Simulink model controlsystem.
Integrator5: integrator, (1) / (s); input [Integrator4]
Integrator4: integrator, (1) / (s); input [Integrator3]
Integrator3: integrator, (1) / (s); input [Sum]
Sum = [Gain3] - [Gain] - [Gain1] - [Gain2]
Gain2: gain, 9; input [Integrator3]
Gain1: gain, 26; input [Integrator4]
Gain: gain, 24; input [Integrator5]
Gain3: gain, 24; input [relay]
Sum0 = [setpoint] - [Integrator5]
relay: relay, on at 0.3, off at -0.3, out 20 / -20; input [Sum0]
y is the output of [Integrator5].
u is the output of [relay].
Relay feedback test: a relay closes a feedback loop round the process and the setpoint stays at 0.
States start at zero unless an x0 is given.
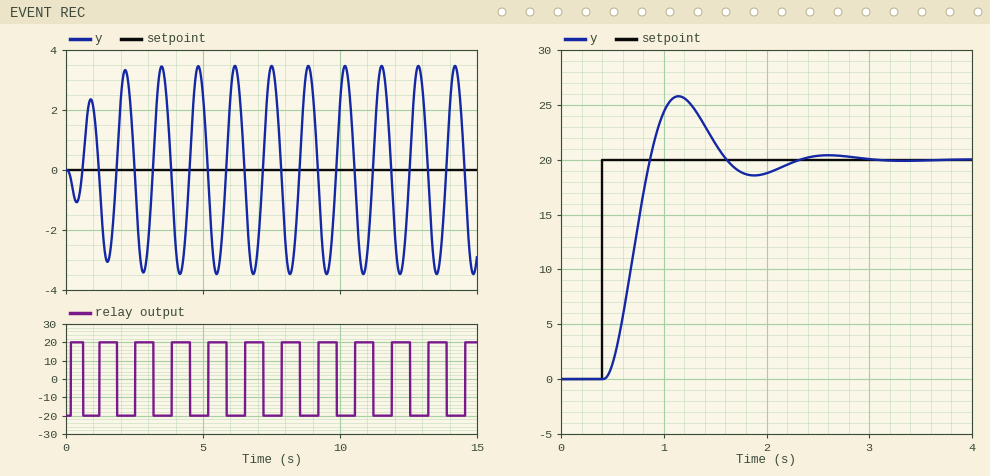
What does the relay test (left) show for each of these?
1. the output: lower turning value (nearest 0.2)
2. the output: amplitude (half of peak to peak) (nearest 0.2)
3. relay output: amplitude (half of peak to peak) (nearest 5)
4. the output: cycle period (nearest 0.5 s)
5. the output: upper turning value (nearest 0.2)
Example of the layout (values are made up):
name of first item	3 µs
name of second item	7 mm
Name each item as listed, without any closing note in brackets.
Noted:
the output: lower turning value	-3.4
the output: amplitude (half of peak to peak)	3.4
relay output: amplitude (half of peak to peak)	20
the output: cycle period	1.5 s
the output: upper turning value	3.4
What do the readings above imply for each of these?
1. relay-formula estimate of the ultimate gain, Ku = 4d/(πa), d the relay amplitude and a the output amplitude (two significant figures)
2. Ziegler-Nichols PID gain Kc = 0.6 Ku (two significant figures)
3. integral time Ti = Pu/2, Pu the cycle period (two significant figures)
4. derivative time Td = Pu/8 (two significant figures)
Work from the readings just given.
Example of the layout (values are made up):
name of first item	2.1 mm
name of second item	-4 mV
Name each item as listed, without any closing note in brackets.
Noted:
relay-formula estimate of the ultimate gain, Ku = 4d/(πa), d the relay amplitude and a the output amplitude	7.5
Ziegler-Nichols PID gain Kc = 0.6 Ku	4.5
integral time Ti = Pu/2, Pu the cycle period	0.75 s
derivative time Td = Pu/8	0.19 s
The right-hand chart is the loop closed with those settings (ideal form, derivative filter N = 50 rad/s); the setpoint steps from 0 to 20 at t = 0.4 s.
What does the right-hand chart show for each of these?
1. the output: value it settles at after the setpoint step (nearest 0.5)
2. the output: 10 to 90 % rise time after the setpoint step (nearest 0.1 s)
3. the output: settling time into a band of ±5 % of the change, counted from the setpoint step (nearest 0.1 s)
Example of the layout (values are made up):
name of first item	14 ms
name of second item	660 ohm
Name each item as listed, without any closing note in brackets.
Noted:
the output: value it settles at after the setpoint step	20.0
the output: 10 to 90 % rise time after the setpoint step	0.3 s
the output: settling time into a band of ±5 % of the change, counted from the setpoint step	1.7 s
